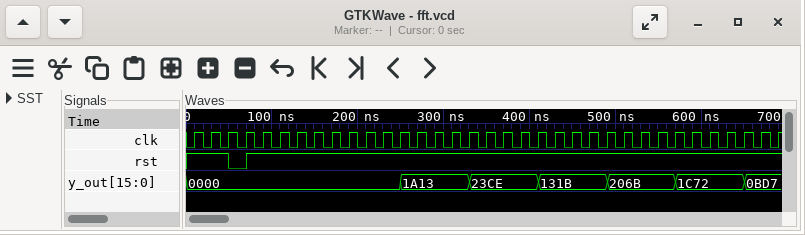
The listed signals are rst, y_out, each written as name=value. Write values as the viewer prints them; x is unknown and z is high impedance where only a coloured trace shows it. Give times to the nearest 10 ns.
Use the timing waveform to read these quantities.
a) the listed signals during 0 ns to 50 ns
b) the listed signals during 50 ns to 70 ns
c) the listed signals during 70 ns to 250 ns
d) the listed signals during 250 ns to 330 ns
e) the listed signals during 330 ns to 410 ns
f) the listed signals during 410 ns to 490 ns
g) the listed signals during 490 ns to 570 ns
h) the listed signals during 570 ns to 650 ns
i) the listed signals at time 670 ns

rst=1, y_out=0000
rst=0, y_out=0000
rst=1, y_out=0000
rst=1, y_out=1A13
rst=1, y_out=23CE
rst=1, y_out=131B
rst=1, y_out=206B
rst=1, y_out=1C72
rst=1, y_out=0BD7
